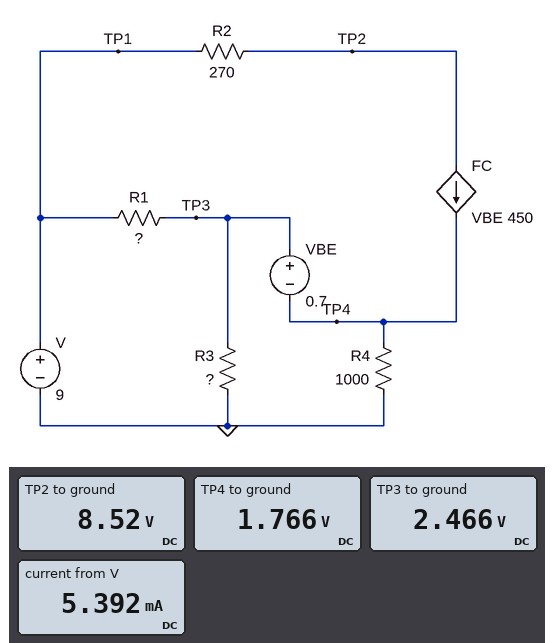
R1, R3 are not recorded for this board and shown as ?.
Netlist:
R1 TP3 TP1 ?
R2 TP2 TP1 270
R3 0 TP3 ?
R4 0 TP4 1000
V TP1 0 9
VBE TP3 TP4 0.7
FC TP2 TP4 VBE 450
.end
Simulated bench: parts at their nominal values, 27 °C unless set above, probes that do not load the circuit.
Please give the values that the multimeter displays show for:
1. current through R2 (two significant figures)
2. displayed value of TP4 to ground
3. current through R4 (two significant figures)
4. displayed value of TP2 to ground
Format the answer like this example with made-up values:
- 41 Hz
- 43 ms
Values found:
- 1.8 mA
- 1.766 V
- 1.8 mA
- 8.52 V
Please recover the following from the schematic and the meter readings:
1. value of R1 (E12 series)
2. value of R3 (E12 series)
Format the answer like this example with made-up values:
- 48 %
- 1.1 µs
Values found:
- 1.8 kΩ
- 680 Ω
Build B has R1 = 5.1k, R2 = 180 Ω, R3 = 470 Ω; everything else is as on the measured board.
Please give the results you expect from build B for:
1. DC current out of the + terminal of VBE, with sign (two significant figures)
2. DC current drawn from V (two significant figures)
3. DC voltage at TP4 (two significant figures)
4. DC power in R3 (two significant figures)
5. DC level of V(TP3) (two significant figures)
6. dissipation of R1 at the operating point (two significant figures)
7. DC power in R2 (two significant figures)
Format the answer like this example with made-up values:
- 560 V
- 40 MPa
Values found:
- -130 nA
- 1.7 mA
- 59 mV
- 1.2 mW
- 760 mV
- 13 mW
- 630 nW
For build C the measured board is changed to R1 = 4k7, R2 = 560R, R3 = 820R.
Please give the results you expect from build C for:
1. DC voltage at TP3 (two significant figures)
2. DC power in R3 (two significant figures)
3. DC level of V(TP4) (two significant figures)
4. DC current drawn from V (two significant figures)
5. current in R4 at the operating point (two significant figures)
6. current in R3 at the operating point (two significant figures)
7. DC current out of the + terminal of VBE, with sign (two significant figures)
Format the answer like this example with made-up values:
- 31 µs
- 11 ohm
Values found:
- 1.3 V
- 2.2 mW
- 640 mV
- 2.3 mA
- 640 µA
- 1.6 mA
- -1.4 µA
